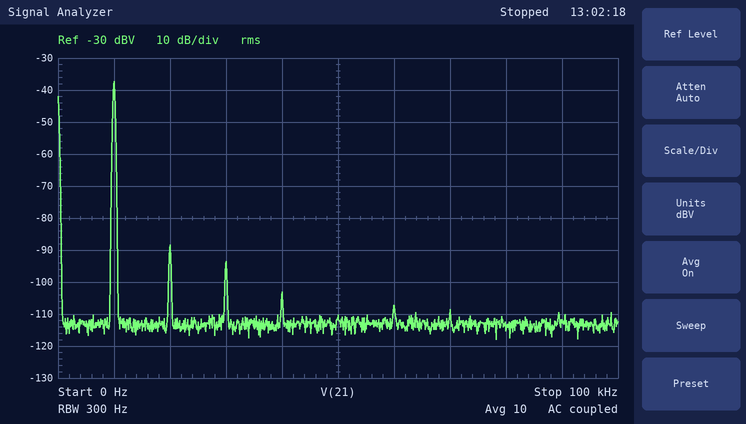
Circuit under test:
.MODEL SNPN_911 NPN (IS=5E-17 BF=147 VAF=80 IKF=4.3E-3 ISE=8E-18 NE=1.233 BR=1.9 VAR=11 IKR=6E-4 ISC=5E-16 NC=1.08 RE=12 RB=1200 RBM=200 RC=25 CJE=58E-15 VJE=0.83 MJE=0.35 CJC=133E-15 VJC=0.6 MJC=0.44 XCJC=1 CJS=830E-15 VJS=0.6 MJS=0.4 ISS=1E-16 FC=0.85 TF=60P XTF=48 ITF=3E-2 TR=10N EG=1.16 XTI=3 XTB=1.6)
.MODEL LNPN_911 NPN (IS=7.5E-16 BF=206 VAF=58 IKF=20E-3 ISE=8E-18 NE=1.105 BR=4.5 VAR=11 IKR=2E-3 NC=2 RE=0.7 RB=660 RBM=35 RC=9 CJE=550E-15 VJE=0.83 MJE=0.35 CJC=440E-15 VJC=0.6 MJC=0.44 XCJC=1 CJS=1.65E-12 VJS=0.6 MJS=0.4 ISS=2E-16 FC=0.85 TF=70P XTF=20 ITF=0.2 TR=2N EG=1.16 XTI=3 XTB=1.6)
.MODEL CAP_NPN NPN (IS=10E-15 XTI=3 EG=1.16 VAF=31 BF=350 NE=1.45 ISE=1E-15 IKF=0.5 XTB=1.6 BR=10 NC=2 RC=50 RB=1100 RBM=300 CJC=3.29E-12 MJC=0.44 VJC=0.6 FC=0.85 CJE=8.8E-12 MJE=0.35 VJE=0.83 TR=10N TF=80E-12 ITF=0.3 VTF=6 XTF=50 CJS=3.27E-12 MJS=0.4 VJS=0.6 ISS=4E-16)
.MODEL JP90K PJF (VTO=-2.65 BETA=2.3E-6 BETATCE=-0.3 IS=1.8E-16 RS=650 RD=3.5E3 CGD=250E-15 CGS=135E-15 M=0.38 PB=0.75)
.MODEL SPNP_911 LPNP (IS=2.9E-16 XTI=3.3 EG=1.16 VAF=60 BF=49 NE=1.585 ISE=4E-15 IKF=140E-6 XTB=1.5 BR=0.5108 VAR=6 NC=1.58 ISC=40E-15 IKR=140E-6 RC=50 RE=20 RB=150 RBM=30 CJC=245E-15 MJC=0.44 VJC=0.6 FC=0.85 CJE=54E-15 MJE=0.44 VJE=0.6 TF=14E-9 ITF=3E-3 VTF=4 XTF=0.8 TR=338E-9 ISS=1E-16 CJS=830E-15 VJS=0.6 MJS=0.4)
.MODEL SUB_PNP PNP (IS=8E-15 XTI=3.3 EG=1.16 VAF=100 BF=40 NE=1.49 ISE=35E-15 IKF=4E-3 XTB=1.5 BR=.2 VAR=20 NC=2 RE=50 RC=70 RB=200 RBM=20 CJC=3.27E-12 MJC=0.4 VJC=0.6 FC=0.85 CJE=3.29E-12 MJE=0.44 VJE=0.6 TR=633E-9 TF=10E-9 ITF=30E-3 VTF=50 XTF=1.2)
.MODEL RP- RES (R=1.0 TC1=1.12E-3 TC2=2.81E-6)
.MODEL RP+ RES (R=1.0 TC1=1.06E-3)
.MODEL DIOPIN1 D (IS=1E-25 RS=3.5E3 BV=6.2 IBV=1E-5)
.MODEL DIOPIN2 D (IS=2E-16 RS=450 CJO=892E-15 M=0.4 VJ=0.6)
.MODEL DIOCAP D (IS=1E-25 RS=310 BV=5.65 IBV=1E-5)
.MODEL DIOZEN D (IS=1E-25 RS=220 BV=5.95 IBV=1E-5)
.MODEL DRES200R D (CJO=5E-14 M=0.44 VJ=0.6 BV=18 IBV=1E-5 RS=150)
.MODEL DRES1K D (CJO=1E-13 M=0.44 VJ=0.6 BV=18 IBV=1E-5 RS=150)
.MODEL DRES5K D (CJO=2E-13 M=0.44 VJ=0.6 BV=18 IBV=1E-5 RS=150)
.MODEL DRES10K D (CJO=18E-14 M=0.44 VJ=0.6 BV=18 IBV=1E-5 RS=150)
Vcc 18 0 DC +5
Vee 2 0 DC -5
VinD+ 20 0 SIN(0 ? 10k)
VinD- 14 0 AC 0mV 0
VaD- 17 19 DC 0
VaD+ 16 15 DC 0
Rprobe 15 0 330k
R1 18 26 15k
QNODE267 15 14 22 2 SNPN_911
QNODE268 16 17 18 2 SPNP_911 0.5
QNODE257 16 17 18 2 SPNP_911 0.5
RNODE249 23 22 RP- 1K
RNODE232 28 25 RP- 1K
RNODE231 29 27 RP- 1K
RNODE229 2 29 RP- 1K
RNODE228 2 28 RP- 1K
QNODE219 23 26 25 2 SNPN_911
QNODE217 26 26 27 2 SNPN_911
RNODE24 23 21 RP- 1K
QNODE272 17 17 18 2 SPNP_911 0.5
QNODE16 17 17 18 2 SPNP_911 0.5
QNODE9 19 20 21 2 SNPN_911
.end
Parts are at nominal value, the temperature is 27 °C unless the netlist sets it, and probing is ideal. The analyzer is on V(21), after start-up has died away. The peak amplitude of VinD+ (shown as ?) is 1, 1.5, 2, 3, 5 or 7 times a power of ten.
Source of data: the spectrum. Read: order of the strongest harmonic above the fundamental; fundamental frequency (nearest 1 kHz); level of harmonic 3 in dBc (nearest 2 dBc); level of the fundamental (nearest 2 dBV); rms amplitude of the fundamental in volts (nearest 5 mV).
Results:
2
10 kHz
-56 dBc
-38 dBV
15 mV
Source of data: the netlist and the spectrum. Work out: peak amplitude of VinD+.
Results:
20 mV
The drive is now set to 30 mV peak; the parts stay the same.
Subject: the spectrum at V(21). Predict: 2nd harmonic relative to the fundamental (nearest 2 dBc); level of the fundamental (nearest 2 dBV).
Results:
-48 dBc
-34 dBV
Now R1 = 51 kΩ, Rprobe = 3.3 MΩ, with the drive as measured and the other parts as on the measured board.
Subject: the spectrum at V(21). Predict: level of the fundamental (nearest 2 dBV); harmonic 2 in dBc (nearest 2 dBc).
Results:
-38 dBV
-40 dBc
